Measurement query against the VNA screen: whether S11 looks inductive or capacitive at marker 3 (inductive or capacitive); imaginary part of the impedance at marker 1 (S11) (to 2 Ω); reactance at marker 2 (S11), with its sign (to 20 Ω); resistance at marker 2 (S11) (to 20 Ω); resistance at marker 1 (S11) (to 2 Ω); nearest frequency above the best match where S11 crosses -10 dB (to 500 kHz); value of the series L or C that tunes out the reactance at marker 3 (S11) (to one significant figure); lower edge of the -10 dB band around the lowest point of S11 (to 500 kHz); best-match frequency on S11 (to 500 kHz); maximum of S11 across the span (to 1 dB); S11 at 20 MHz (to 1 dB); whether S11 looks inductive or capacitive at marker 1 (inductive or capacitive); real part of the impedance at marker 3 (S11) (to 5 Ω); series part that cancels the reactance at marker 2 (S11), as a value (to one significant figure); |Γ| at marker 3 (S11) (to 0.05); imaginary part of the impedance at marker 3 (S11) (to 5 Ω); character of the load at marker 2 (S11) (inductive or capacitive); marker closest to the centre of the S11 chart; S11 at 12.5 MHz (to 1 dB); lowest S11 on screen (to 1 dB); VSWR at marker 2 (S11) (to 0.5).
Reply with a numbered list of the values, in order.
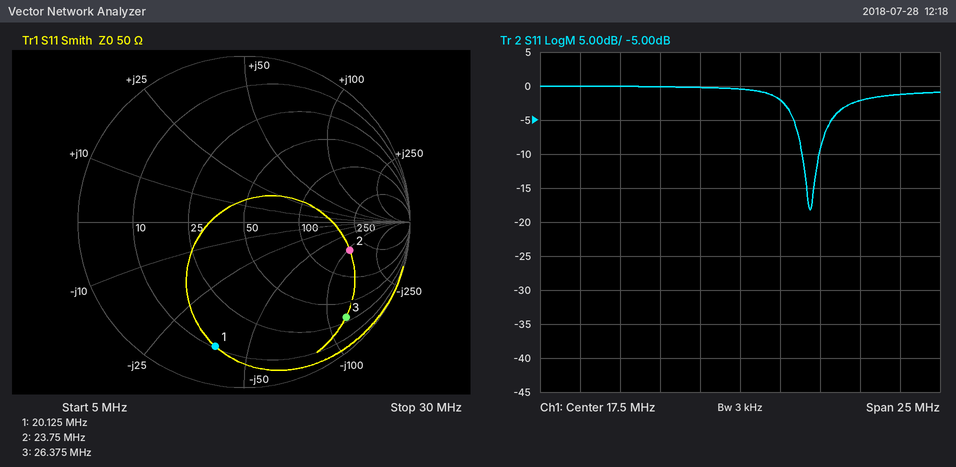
1. capacitive
2. -38 Ω
3. -100 Ω
4. 180 Ω
5. 10 Ω
6. 22.5 MHz
7. 700 nH
8. 21.5 MHz
9. 22.0 MHz
10. 0 dB
11. -2 dB
12. capacitive
13. 30 Ω
14. 700 nH
15. 0.85
16. -120 Ω
17. capacitive
18. marker 2
19. 0 dB
20. -18 dB
21. 5.0
